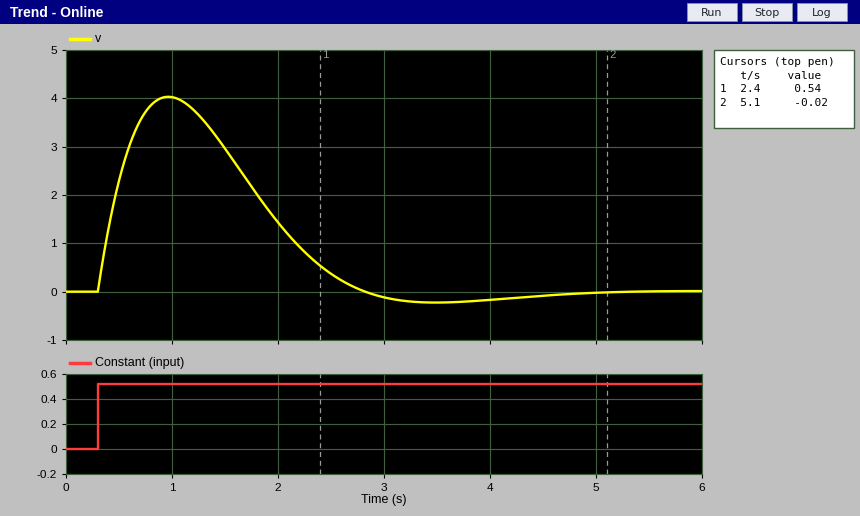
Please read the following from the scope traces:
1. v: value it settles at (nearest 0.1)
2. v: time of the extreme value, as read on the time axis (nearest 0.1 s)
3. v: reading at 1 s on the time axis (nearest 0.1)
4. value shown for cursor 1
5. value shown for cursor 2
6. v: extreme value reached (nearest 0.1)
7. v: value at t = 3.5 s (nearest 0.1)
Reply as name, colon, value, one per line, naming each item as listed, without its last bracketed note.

v: value it settles at: 0.0
v: time of the extreme value, as read on the time axis: 1.0 s
v: reading at 1 s on the time axis: 4.0
value shown for cursor 1: 0.54
value shown for cursor 2: -0.02
v: extreme value reached: 4.0
v: value at t = 3.5 s: -0.2
